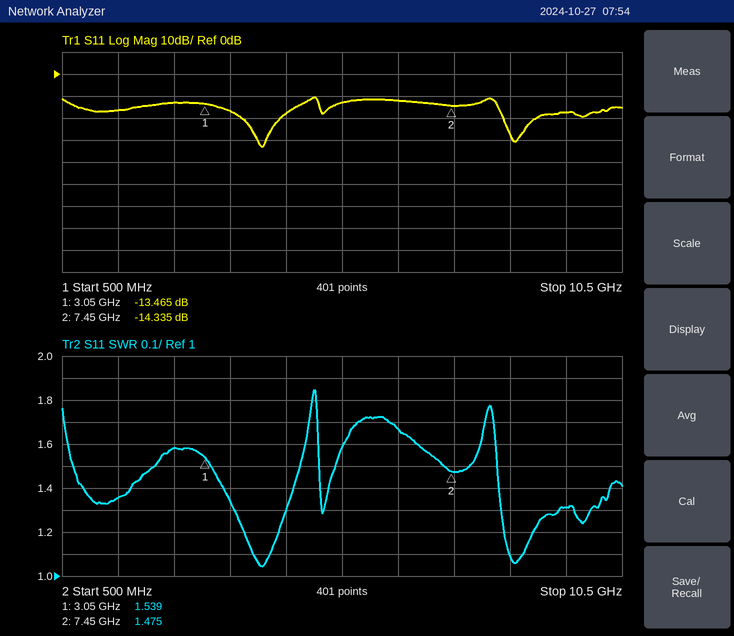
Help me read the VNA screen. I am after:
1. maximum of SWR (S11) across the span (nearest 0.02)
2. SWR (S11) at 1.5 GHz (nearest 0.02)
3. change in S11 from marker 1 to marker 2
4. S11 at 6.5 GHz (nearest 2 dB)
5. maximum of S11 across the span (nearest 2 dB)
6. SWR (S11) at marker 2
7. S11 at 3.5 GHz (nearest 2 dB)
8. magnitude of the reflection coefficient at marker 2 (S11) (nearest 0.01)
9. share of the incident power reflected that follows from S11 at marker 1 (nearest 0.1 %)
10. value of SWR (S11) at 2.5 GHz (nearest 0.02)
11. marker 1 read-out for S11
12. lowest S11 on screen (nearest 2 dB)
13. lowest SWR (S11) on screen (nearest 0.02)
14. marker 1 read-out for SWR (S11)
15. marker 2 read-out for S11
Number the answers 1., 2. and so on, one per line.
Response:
1. 1.84
2. 1.36
3. -0.870 dB
4. -12 dB
5. -10 dB
6. 1.475
7. -16 dB
8. 0.19
9. 4.5 %
10. 1.58
11. -13.465 dB
12. -34 dB
13. 1.04
14. 1.539
15. -14.335 dB
